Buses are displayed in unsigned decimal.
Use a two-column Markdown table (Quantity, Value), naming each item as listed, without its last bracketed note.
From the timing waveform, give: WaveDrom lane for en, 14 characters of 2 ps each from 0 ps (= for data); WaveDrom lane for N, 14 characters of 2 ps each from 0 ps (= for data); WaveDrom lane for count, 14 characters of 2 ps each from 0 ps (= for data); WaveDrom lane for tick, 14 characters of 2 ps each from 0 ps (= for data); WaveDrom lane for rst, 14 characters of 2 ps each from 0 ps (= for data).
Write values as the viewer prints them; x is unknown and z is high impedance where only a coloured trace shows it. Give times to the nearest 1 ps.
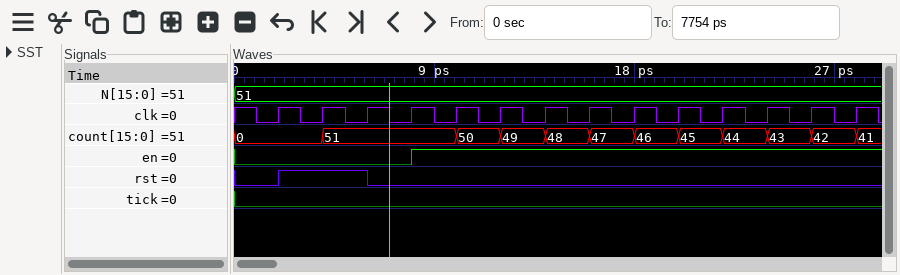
| Quantity | Value |
|---|---|
| WaveDrom lane for en, 14 characters of 2 ps each from 0 ps | {name: 'en', wave: '0...1.........'} |
| WaveDrom lane for N, 14 characters of 2 ps each from 0 ps | {name: 'N', wave: '=.............', data: '51'} |
| WaveDrom lane for count, 14 characters of 2 ps each from 0 ps | {name: 'count', wave: '=.=..=========', data: '0 51 50 49 48 47 46 45 44 43 42'} |
| WaveDrom lane for tick, 14 characters of 2 ps each from 0 ps | {name: 'tick', wave: '0.............'} |
| WaveDrom lane for rst, 14 characters of 2 ps each from 0 ps | {name: 'rst', wave: '01.0..........'} |
